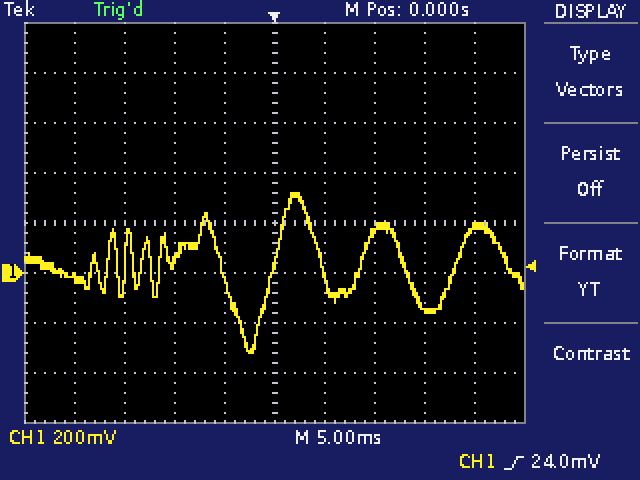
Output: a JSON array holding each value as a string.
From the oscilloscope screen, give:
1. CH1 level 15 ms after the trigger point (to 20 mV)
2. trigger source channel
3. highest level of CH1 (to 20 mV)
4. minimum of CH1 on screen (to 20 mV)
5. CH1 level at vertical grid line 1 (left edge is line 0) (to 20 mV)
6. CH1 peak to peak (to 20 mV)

["-140 mV", "CH1", "320 mV", "-320 mV", "-20 mV", "640 mV"]
